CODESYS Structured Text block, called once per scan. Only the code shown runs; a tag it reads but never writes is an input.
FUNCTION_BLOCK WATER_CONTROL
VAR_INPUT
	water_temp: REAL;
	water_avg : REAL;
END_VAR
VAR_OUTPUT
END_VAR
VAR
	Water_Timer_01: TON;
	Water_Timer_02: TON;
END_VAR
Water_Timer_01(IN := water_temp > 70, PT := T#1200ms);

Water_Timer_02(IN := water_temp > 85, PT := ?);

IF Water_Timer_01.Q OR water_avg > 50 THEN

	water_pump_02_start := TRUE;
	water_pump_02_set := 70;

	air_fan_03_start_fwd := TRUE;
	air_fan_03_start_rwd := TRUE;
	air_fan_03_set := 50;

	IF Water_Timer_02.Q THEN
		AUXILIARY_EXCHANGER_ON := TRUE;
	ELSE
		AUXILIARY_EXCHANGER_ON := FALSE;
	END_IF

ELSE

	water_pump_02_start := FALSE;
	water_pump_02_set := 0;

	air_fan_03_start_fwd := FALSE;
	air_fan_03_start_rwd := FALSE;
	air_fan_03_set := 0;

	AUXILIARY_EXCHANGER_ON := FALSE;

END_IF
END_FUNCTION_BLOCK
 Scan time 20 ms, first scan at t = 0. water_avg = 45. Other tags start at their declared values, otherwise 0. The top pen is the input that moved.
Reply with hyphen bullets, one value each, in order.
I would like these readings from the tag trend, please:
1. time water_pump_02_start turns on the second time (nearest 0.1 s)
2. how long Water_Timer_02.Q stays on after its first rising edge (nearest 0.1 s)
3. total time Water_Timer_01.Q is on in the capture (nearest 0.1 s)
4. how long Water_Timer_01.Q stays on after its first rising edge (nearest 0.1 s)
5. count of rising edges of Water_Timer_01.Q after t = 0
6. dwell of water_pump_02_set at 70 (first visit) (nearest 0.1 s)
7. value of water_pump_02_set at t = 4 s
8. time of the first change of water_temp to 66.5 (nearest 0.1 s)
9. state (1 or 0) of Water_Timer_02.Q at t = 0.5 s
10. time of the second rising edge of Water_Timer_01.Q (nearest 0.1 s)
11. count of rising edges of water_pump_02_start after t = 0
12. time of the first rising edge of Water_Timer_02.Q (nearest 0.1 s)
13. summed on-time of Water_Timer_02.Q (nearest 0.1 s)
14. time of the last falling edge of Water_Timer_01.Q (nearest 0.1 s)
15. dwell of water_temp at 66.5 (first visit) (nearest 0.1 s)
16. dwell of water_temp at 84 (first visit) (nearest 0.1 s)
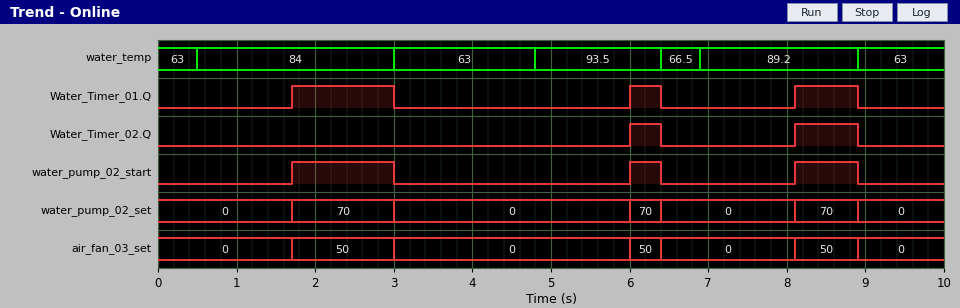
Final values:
- 6.0 s
- 0.4 s
- 2.5 s
- 1.3 s
- 3
- 1.3 s
- 0
- 6.4 s
- 0
- 6.0 s
- 3
- 6.0 s
- 1.2 s
- 8.9 s
- 0.5 s
- 2.5 s
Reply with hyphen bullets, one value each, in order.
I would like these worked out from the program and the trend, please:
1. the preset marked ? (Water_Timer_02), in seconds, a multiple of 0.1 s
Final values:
- 1.2 s
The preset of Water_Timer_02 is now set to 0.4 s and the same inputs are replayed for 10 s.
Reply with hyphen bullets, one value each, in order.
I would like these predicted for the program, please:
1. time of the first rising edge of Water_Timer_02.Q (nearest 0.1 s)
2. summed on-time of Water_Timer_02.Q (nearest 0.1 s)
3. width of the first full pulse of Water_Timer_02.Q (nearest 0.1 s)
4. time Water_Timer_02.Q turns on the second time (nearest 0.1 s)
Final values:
- 5.2 s
- 2.8 s
- 1.2 s
- 7.3 s
